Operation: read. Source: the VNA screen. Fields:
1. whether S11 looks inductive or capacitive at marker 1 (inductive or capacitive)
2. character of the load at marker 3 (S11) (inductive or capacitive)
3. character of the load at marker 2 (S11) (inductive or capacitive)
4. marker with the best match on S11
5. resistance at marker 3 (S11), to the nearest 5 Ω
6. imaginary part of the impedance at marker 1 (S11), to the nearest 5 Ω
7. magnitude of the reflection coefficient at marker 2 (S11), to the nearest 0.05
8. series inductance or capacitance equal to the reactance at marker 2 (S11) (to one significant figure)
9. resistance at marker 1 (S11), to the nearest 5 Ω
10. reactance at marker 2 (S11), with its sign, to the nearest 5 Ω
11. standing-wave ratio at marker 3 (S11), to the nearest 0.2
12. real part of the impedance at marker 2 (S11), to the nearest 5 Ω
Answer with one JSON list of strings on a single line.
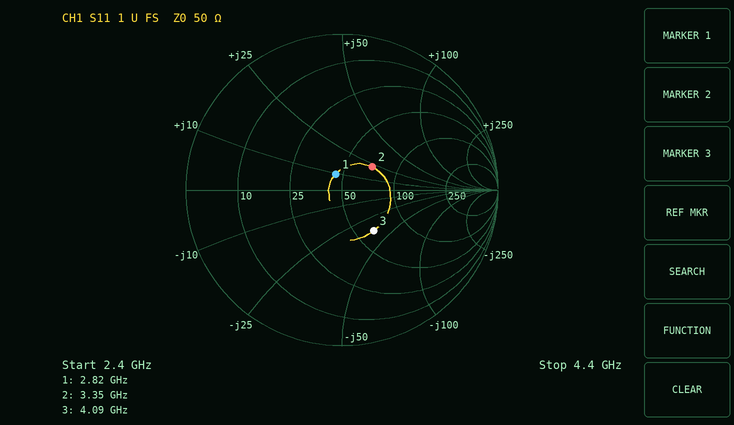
["inductive", "capacitive", "inductive", "marker 1", "65 Ω", "+10 Ω", "0.25", "1 nH", "45 Ω", "+20 Ω", "2.0", "70 Ω"]
